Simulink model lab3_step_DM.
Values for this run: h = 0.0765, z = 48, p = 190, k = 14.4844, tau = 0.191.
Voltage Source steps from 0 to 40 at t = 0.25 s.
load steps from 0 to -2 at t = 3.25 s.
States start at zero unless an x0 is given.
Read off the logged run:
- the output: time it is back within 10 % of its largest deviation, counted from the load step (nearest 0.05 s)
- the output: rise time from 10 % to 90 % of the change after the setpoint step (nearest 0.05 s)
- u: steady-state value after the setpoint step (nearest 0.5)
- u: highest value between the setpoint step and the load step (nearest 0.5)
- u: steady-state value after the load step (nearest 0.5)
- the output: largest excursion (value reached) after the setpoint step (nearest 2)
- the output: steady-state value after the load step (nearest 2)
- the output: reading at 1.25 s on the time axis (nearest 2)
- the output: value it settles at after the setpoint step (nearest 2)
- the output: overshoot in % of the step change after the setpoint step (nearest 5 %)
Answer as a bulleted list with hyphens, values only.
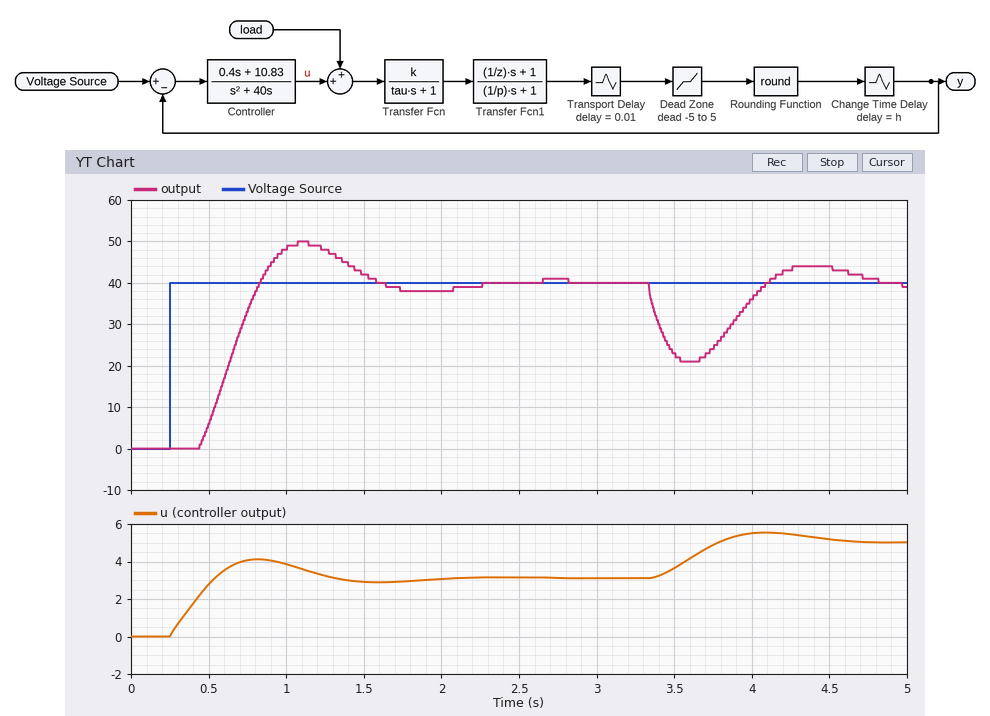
- 1.45 s
- 0.30 s
- 3.0
- 4.0
- 5.0
- 50
- 40
- 48
- 40
- 25 %
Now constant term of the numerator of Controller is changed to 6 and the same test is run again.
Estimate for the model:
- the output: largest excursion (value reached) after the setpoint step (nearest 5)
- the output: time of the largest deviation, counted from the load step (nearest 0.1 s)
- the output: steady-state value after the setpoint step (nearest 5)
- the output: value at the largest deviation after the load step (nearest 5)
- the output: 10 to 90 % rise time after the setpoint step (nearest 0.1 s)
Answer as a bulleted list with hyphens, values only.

- 40
- 0.3 s
- 40
- 20
- 0.6 s
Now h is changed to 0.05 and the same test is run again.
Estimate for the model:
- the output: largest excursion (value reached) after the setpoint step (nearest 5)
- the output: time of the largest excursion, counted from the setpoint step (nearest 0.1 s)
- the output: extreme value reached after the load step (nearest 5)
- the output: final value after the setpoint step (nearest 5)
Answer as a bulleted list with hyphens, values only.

- 45
- 0.8 s
- 20
- 40
